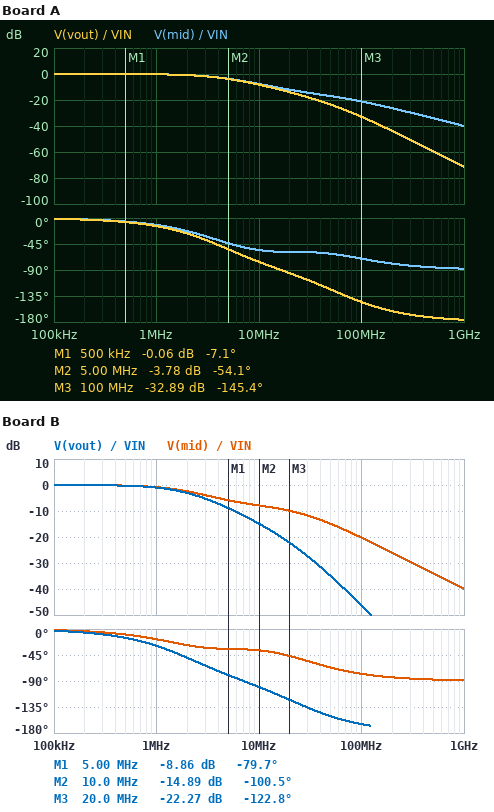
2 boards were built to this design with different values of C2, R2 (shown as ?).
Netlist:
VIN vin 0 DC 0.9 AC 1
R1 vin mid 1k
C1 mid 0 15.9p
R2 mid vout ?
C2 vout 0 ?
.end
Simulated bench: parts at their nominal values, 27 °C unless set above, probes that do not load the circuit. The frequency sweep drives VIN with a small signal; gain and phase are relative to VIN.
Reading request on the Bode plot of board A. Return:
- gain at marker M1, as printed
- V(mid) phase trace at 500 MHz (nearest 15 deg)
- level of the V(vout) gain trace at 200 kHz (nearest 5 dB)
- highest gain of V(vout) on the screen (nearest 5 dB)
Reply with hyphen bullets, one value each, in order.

- -0.06 dB
- -90 deg
- 0 dB
- 0 dB
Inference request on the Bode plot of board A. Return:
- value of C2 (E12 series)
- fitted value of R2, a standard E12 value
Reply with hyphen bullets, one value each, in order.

- 18 pF
- 330 Ω
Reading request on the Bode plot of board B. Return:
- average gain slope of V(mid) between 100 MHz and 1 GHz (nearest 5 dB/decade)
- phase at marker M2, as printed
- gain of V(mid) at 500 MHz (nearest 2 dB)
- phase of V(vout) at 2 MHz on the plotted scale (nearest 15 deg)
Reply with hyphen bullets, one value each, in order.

- -20 dB/decade
- -100.5 deg
- -34 dB
- -45 deg
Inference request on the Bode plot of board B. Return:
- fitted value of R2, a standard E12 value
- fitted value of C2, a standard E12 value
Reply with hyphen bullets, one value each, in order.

- 820 Ω
- 39 pF
